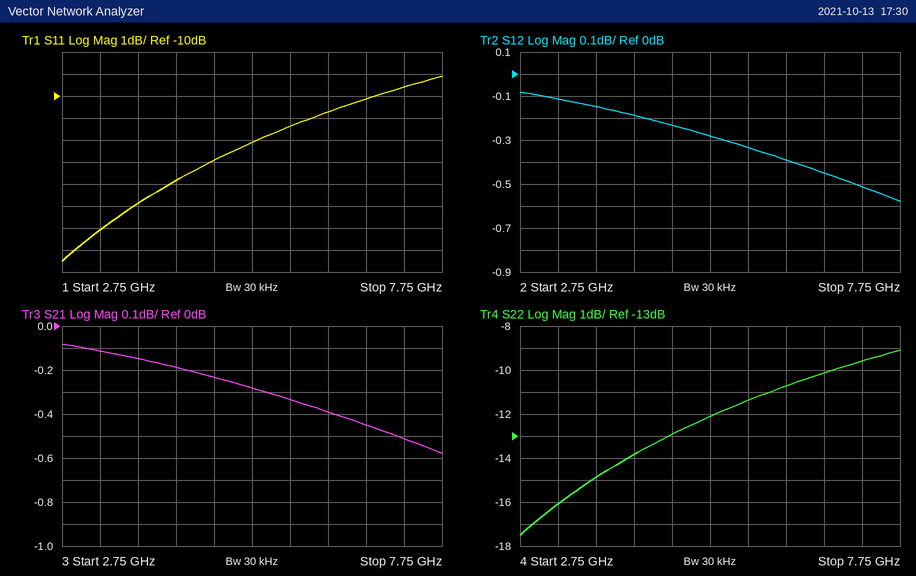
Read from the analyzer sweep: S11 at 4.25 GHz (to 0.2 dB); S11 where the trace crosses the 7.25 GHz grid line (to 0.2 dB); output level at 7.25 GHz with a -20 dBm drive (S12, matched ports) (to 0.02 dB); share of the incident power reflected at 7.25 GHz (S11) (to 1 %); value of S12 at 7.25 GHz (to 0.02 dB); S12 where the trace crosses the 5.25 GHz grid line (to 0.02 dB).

-13.8 dB
-9.6 dB
-20.52 dBm
11 %
-0.52 dB
-0.28 dB
